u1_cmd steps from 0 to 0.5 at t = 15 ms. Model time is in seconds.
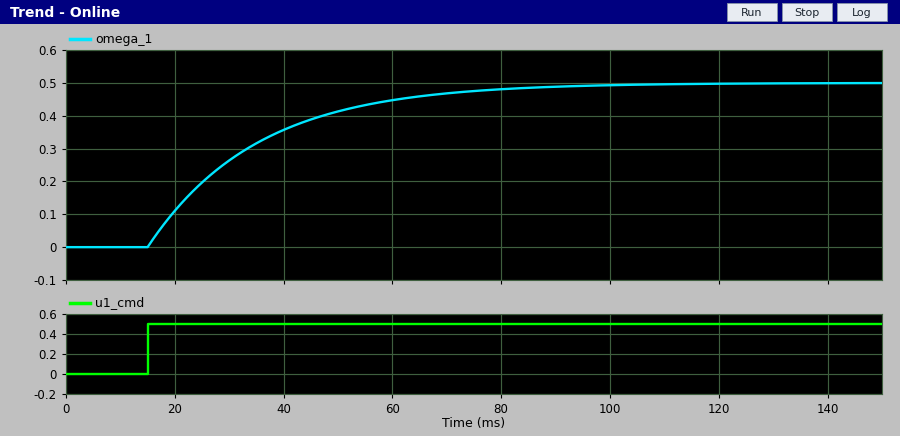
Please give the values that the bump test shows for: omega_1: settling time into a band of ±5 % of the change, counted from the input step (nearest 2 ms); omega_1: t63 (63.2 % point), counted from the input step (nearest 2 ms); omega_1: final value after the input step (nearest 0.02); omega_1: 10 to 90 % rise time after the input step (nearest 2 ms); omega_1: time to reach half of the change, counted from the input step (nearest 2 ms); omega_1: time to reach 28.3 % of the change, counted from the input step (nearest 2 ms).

60 ms
20 ms
0.50
44 ms
14 ms
6 ms
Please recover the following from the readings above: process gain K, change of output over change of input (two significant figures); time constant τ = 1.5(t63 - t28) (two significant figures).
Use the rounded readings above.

1.0
21 ms
